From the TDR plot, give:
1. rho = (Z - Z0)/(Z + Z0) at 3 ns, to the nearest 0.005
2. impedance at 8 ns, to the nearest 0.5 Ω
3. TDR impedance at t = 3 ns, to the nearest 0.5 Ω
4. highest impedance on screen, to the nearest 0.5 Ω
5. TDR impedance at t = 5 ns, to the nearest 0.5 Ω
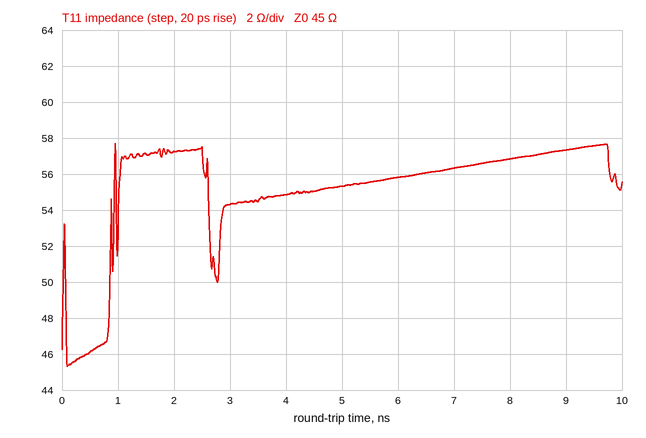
+0.095
57.0 Ω
54.5 Ω
57.5 Ω
55.5 Ω
